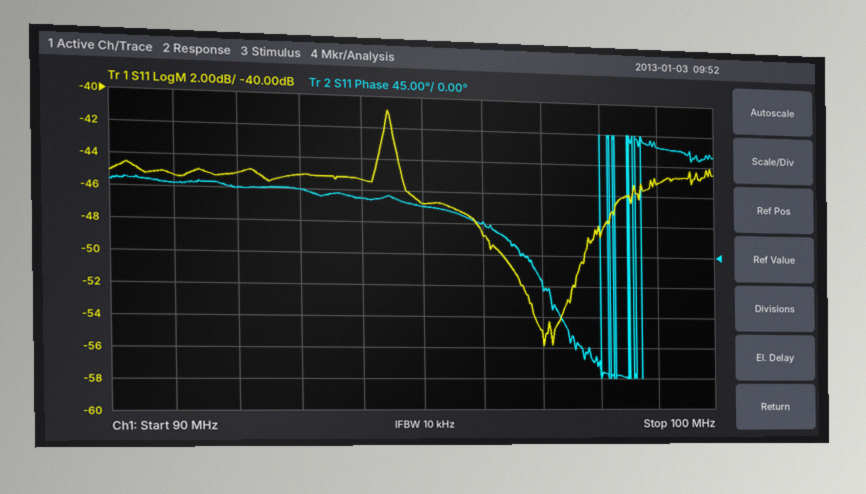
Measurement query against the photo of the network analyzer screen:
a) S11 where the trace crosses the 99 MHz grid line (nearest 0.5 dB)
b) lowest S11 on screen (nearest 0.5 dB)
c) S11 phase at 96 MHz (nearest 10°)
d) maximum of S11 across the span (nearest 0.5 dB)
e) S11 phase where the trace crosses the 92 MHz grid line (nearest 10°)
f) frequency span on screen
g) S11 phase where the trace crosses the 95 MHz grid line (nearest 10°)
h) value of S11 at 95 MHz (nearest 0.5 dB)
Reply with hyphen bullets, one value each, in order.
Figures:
- -45.0 dB
- -56.0 dB
- 50°
- -41.0 dB
- 90°
- 10 MHz
- 70°
- -47.0 dB
